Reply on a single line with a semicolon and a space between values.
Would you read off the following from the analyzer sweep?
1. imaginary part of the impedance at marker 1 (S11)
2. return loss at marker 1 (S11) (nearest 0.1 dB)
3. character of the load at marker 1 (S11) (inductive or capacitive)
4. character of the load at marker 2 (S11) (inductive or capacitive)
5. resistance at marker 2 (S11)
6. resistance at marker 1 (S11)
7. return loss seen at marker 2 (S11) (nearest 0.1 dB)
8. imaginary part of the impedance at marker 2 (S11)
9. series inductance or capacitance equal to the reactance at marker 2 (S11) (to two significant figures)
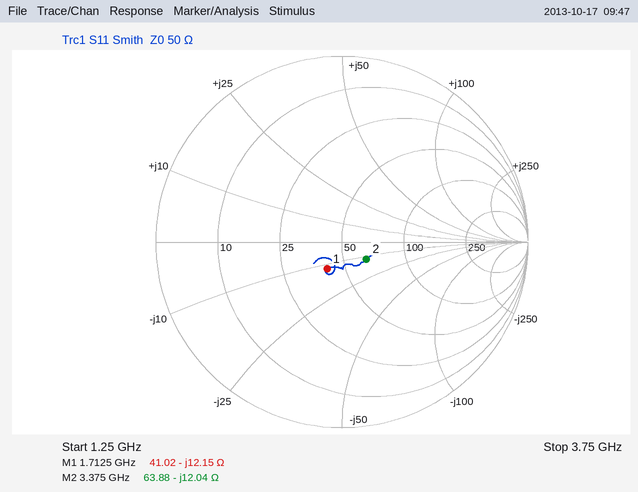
-12.15 Ω; 15.7 dB; capacitive; capacitive; 63.88 Ω; 41.02 Ω; 15.9 dB; -12.04 Ω; 3.9 pF
